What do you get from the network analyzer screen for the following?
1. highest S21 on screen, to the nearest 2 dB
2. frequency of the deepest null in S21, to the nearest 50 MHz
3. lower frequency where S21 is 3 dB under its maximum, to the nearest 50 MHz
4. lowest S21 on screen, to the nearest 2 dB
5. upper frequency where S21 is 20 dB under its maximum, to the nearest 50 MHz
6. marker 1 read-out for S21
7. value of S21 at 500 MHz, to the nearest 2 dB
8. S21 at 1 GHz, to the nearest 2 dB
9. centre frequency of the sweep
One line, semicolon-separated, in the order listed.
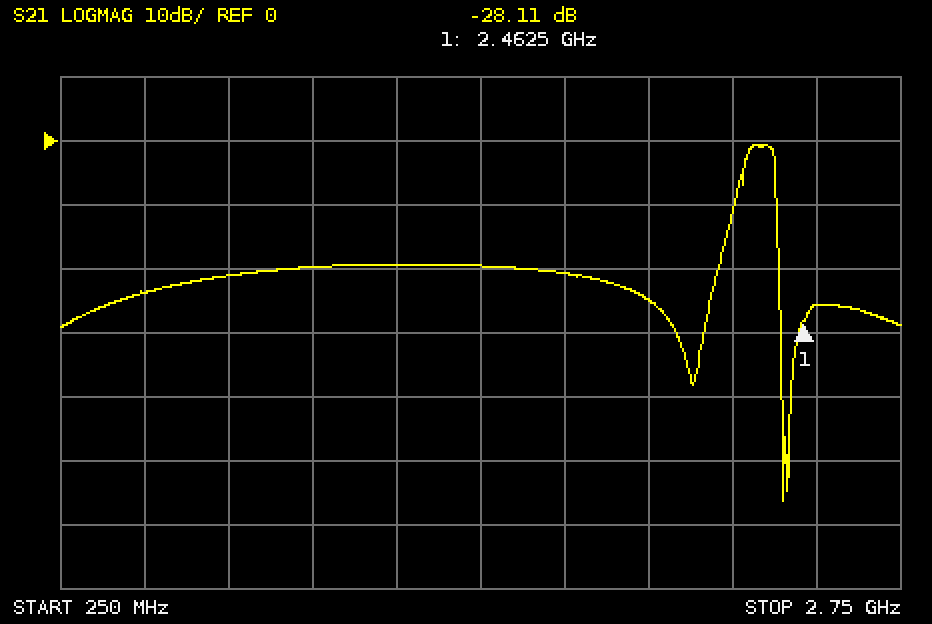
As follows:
0 dB; 2.40 GHz; 2.30 GHz; -56 dB; 2.40 GHz; -28.11 dB; -24 dB; -20 dB; 1.5 GHz
